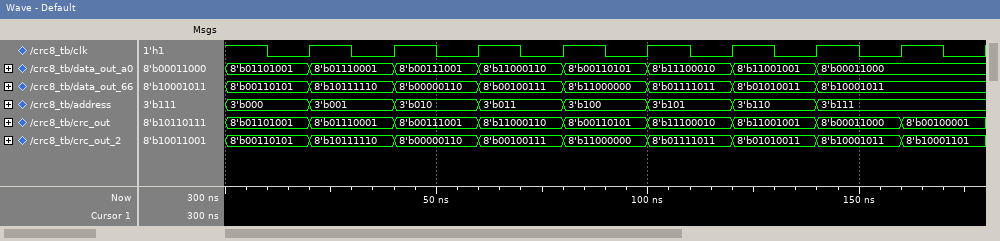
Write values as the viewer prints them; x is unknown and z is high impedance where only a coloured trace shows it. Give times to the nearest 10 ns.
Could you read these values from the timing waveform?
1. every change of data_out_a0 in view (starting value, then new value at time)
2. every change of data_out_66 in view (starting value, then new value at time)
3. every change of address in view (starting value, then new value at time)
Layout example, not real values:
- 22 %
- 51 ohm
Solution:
- 8'b01101001, 8'b01110001 at 20 ns, 8'b00111001 at 40 ns, 8'b11000110 at 60 ns, 8'b00110101 at 80 ns, 8'b11100010 at 100 ns, 8'b11001001 at 120 ns, 8'b00011000 at 140 ns
- 8'b00110101, 8'b10111110 at 20 ns, 8'b00000110 at 40 ns, 8'b00100111 at 60 ns, 8'b11000000 at 80 ns, 8'b01111011 at 100 ns, 8'b01010011 at 120 ns, 8'b10001011 at 140 ns
- 3'b000, 3'b001 at 20 ns, 3'b010 at 40 ns, 3'b011 at 60 ns, 3'b100 at 80 ns, 3'b101 at 100 ns, 3'b110 at 120 ns, 3'b111 at 140 ns
